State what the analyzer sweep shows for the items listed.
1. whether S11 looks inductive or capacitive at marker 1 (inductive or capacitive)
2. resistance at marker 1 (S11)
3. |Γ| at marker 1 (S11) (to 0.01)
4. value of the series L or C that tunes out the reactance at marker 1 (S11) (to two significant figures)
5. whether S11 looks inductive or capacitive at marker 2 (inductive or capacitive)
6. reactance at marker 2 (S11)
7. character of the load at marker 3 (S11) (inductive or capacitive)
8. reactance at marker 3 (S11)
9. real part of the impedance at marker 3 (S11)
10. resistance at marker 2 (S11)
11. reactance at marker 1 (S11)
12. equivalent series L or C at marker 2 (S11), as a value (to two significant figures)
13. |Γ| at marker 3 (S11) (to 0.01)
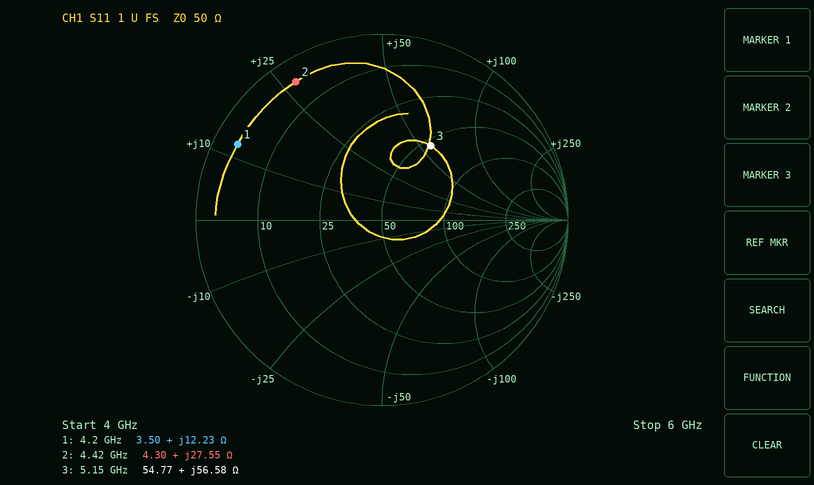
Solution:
inductive
3.50 Ω
0.88
3.1 pF
inductive
+27.55 Ω
inductive
+56.58 Ω
54.77 Ω
4.30 Ω
+12.23 Ω
990 pH
0.48
